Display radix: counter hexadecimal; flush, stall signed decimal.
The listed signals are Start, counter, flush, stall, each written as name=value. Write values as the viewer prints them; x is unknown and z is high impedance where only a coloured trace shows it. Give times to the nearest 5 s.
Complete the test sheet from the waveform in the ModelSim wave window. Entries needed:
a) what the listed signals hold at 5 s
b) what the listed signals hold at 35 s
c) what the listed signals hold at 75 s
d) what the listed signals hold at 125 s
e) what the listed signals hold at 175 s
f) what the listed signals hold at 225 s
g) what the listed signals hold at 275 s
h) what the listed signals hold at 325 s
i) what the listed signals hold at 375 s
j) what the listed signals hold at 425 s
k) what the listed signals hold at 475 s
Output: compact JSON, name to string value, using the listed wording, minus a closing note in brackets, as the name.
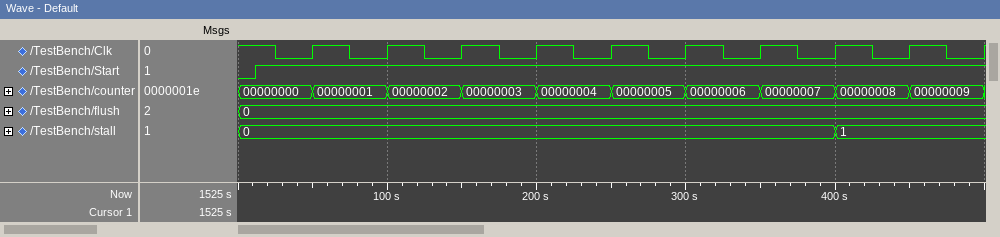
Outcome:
{"what the listed signals hold at 5 s": "Start=0, counter=00000000, flush=0, stall=0", "what the listed signals hold at 35 s": "Start=1, counter=00000000, flush=0, stall=0", "what the listed signals hold at 75 s": "Start=1, counter=00000001, flush=0, stall=0", "what the listed signals hold at 125 s": "Start=1, counter=00000002, flush=0, stall=0", "what the listed signals hold at 175 s": "Start=1, counter=00000003, flush=0, stall=0", "what the listed signals hold at 225 s": "Start=1, counter=00000004, flush=0, stall=0", "what the listed signals hold at 275 s": "Start=1, counter=00000005, flush=0, stall=0", "what the listed signals hold at 325 s": "Start=1, counter=00000006, flush=0, stall=0", "what the listed signals hold at 375 s": "Start=1, counter=00000007, flush=0, stall=0", "what the listed signals hold at 425 s": "Start=1, counter=00000008, flush=0, stall=1", "what the listed signals hold at 475 s": "Start=1, counter=00000009, flush=0, stall=1"}
